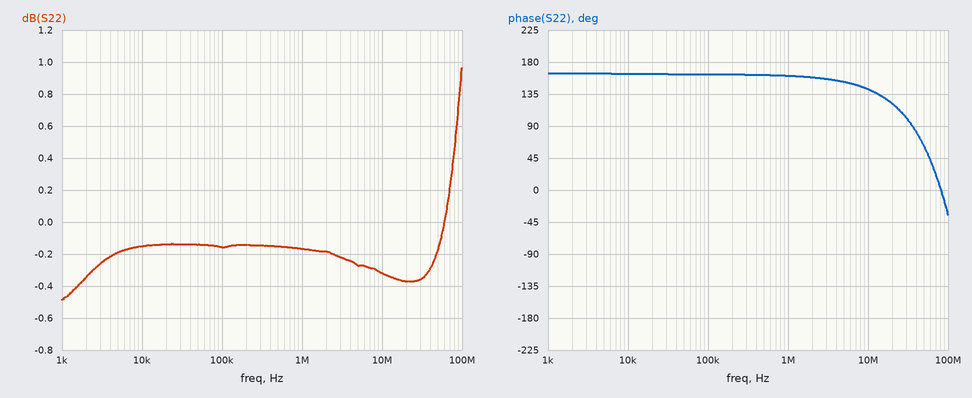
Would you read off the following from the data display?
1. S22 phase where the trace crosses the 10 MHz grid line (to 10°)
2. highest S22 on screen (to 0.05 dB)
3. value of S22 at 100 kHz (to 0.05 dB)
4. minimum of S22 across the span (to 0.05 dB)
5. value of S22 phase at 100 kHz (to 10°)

140°
0.95 dB
-0.15 dB
-0.50 dB
160°
